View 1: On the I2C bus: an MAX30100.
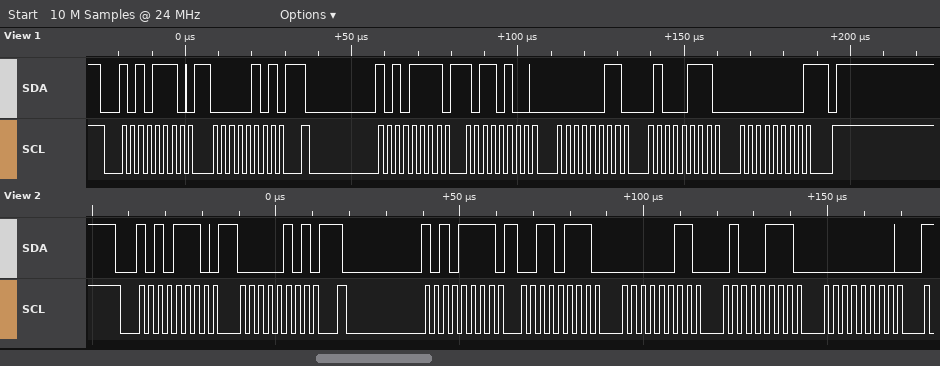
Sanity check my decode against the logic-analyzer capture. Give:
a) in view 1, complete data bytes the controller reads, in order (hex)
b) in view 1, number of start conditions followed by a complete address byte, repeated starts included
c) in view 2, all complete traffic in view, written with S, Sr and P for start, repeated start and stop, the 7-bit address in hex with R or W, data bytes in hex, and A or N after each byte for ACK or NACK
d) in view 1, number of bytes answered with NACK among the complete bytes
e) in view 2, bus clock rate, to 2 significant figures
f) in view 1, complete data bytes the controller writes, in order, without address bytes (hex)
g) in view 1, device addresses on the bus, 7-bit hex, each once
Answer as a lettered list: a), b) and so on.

a) B4 03 47 00
b) 2
c) S 57W A 05 A Sr 57R A 37 A 03 A 47 A 00 A
d) 1
e) 400 kHz
f) 05
g) 0x57
